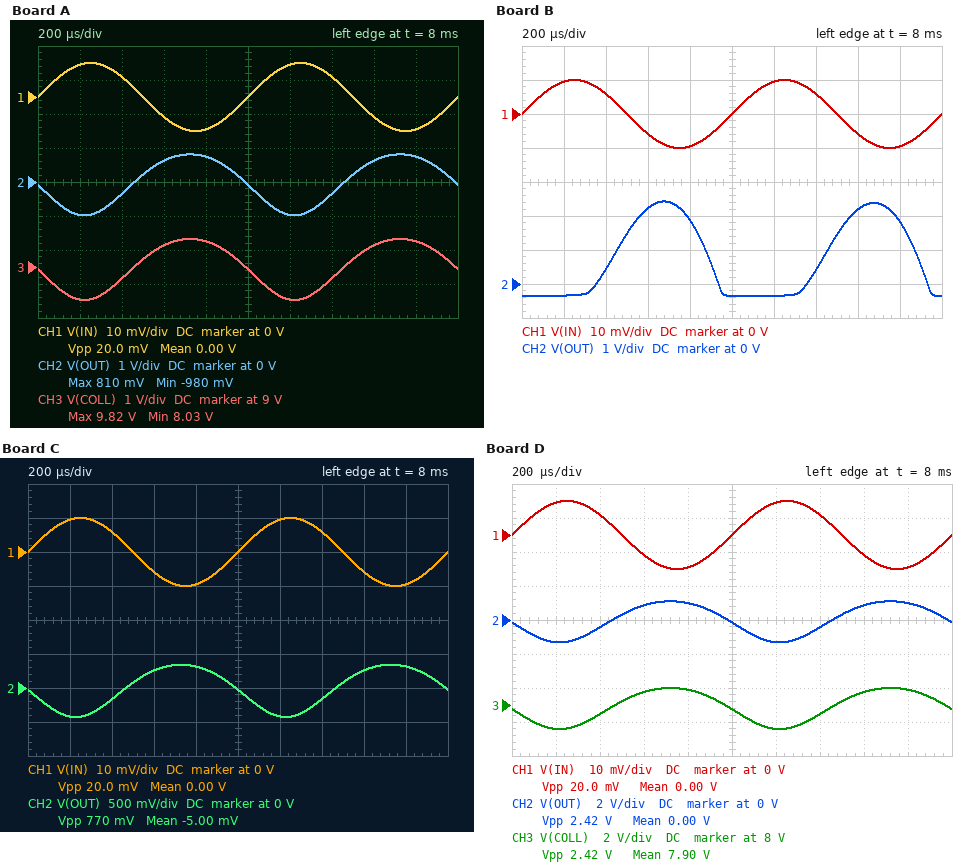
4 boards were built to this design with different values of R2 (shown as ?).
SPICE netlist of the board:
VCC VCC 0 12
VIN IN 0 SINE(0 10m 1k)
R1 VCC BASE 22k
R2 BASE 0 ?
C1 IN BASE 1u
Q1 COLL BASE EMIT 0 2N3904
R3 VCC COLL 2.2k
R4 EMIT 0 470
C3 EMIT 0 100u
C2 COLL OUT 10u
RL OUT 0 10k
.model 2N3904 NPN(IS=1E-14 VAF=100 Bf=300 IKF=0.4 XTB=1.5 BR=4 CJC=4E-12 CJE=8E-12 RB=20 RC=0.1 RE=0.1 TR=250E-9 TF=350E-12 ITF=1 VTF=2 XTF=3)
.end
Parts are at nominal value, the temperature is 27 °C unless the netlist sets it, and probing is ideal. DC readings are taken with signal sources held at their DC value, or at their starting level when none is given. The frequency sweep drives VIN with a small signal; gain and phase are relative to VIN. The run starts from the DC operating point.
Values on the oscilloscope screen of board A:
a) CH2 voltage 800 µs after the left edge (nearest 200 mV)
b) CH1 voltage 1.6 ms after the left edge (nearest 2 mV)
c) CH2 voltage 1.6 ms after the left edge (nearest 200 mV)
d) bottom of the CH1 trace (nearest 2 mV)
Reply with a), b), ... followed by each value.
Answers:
a) 800 mV
b) -6 mV
c) 600 mV
d) -10 mV
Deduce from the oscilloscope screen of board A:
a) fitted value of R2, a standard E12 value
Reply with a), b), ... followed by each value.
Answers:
a) 2.7 kΩ
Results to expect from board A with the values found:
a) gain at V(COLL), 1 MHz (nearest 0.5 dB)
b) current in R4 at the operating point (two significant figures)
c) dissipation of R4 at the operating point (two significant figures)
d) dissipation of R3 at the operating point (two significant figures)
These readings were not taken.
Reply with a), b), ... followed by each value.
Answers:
a) 39.0 dB
b) 1.4 mA
c) 870 µW
d) 4.1 mW
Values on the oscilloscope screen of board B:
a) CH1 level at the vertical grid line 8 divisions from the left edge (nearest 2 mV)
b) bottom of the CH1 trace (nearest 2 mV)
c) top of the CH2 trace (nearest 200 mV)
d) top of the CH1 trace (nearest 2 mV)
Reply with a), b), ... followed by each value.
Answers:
a) -6 mV
b) -10 mV
c) 2.4 V
d) 10 mV
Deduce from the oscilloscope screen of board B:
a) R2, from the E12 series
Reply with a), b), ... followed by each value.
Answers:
a) 6.8 kΩ
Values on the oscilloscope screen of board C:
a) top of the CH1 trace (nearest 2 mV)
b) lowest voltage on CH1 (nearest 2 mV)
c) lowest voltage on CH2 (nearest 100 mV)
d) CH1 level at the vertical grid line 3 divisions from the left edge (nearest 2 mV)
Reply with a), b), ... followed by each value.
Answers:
a) 10 mV
b) -10 mV
c) -400 mV
d) -6 mV
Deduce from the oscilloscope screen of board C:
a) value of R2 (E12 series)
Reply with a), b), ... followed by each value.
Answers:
a) 1.8 kΩ
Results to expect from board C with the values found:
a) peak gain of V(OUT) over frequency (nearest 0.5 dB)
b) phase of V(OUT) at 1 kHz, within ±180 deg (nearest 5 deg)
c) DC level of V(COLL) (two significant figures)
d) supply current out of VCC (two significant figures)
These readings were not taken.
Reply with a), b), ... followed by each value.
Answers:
a) 32.0 dB
b) -170 deg
c) 11 V
d) 1.1 mA
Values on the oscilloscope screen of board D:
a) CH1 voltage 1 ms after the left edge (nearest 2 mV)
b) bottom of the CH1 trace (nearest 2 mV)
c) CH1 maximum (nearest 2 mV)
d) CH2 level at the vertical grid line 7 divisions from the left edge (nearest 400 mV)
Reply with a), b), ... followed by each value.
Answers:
a) 0 V
b) -10 mV
c) 10 mV
d) -400 mV
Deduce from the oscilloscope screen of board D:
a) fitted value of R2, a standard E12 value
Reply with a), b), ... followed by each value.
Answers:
a) 3.3 kΩ
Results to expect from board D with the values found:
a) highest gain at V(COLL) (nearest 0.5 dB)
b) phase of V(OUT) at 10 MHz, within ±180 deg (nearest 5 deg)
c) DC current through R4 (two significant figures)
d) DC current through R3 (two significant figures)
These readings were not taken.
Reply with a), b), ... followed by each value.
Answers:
a) 42.0 dB
b) 150 deg
c) 1.9 mA
d) 1.9 mA
